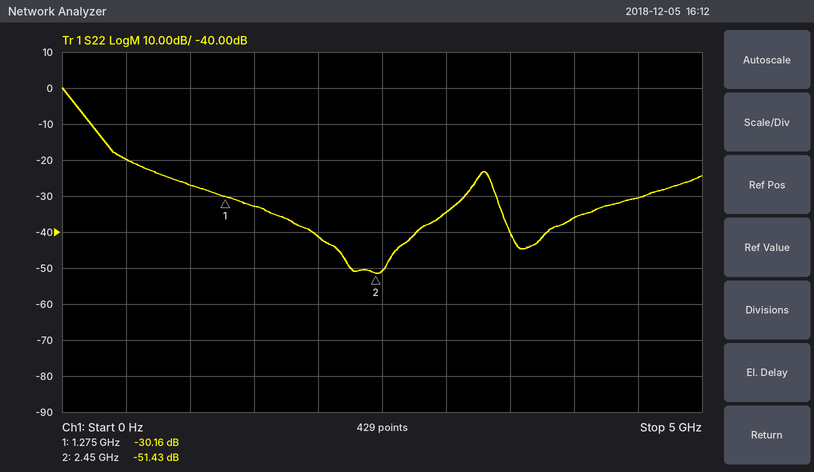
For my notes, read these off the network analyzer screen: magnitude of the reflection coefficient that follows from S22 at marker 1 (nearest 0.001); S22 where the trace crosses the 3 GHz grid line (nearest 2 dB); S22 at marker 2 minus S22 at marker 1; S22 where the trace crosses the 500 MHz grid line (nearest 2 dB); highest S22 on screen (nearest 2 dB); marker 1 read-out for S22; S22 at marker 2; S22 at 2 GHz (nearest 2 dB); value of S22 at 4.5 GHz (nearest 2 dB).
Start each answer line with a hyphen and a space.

- 0.031
- -34 dB
- -21.27 dB
- -20 dB
- 0 dB
- -30.16 dB
- -51.43 dB
- -42 dB
- -30 dB
